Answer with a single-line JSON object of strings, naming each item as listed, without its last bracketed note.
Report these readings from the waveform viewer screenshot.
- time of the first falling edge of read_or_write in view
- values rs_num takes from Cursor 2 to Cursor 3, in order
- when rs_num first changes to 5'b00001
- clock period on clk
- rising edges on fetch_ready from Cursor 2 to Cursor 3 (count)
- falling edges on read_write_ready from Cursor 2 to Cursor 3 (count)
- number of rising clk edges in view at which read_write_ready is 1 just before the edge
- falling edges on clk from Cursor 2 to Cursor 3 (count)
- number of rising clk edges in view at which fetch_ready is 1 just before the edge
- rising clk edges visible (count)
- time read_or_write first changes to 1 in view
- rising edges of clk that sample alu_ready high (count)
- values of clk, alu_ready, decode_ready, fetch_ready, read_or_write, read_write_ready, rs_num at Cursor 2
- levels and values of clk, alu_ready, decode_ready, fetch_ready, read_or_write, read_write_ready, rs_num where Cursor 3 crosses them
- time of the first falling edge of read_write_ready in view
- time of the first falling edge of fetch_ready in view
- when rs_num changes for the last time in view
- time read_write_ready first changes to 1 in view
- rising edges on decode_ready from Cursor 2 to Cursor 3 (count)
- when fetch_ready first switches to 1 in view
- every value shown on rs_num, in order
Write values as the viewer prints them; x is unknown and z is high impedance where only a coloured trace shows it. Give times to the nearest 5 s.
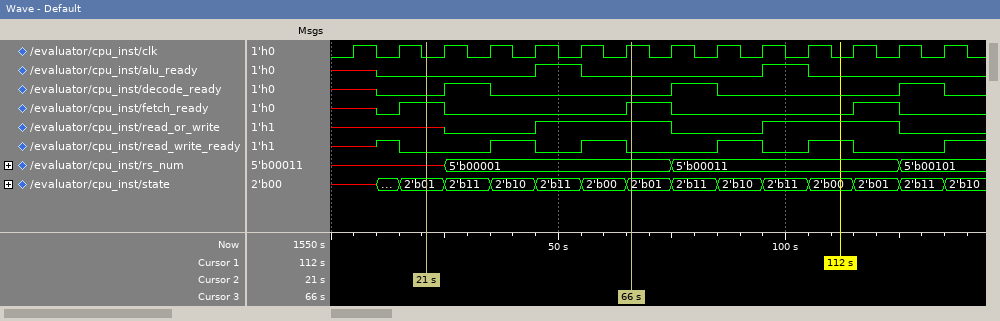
{"time of the first falling edge of read_or_write in view": "75 s", "values rs_num takes from Cursor 2 to Cursor 3, in order": "x, 5'b00001", "when rs_num first changes to 5'b00001": "25 s", "clock period on clk": "10 s", "rising edges on fetch_ready from Cursor 2 to Cursor 3": "1", "falling edges on read_write_ready from Cursor 2 to Cursor 3": "2", "number of rising clk edges in view at which read_write_ready is 1 just before the edge": "5", "falling edges on clk from Cursor 2 to Cursor 3": "4", "number of rising clk edges in view at which fetch_ready is 1 just before the edge": "3", "rising clk edges visible": "14", "time read_or_write first changes to 1 in view": "45 s", "rising edges of clk that sample alu_ready high": "2", "values of clk, alu_ready, decode_ready, fetch_ready, read_or_write, read_write_ready, rs_num at Cursor 2": "clk=0, alu_ready=0, decode_ready=0, fetch_ready=1, read_or_write=x, read_write_ready=0, rs_num=x", "levels and values of clk, alu_ready, decode_ready, fetch_ready, read_or_write, read_write_ready, rs_num where Cursor 3 crosses them": "clk=1, alu_ready=0, decode_ready=0, fetch_ready=1, read_or_write=1, read_write_ready=0, rs_num=5'b00001", "time of the first falling edge of read_write_ready in view": "15 s", "time of the first falling edge of fetch_ready in view": "25 s", "when rs_num changes for the last time in view": "125 s", "time read_write_ready first changes to 1 in view": "10 s", "rising edges on decode_ready from Cursor 2 to Cursor 3": "1", "when fetch_ready first switches to 1 in view": "15 s", "every value shown on rs_num, in order": "x, 5'b00001, 5'b00011, 5'b00101"}
